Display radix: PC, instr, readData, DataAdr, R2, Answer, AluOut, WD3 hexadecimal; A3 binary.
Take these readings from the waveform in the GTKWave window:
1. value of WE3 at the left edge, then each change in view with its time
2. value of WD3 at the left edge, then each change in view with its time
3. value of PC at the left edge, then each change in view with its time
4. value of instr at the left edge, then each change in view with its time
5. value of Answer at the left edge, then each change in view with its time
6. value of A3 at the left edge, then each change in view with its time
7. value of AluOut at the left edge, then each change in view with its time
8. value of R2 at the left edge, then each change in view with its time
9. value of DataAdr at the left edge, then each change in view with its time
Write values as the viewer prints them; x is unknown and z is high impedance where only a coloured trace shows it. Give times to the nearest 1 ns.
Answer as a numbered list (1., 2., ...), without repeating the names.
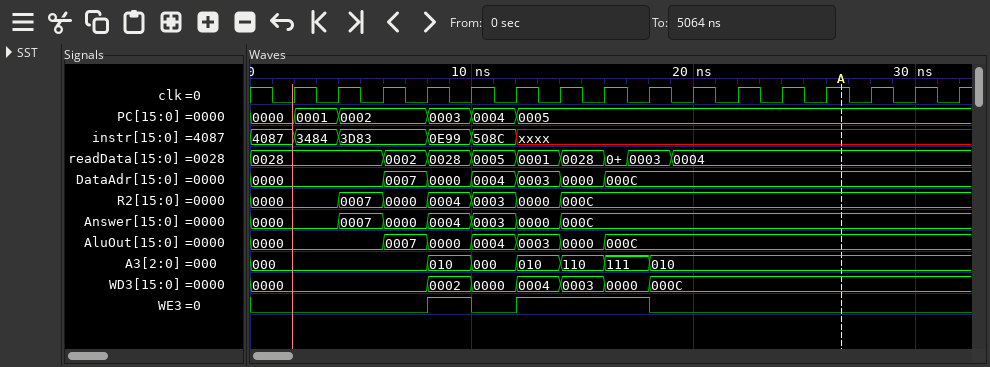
1. 0, 1 at 8 ns, 0 at 10 ns, 1 at 12 ns, 0 at 18 ns
2. 0000, 0002 at 8 ns, 0000 at 10 ns, 0004 at 12 ns, 0003 at 14 ns, 0000 at 16 ns, 000C at 18 ns
3. 0000, 0001 at 2 ns, 0002 at 4 ns, 0003 at 8 ns, 0004 at 10 ns, 0005 at 12 ns
4. 4087, 3484 at 2 ns, 3D83 at 4 ns, 0E99 at 8 ns, 508C at 10 ns, xxxx at 12 ns
5. 0000, 0007 at 4 ns, 0000 at 6 ns, 0004 at 8 ns, 0003 at 10 ns, 0000 at 12 ns, 000C at 14 ns
6. 000, 010 at 8 ns, 000 at 10 ns, 010 at 12 ns, 110 at 14 ns, 111 at 16 ns, 010 at 18 ns
7. 0000, 0007 at 6 ns, 0000 at 8 ns, 0004 at 10 ns, 0003 at 12 ns, 0000 at 14 ns, 000C at 16 ns
8. 0000, 0007 at 4 ns, 0000 at 6 ns, 0004 at 8 ns, 0003 at 10 ns, 0000 at 12 ns, 000C at 14 ns
9. 0000, 0007 at 6 ns, 0000 at 8 ns, 0004 at 10 ns, 0003 at 12 ns, 0000 at 14 ns, 000C at 16 ns
